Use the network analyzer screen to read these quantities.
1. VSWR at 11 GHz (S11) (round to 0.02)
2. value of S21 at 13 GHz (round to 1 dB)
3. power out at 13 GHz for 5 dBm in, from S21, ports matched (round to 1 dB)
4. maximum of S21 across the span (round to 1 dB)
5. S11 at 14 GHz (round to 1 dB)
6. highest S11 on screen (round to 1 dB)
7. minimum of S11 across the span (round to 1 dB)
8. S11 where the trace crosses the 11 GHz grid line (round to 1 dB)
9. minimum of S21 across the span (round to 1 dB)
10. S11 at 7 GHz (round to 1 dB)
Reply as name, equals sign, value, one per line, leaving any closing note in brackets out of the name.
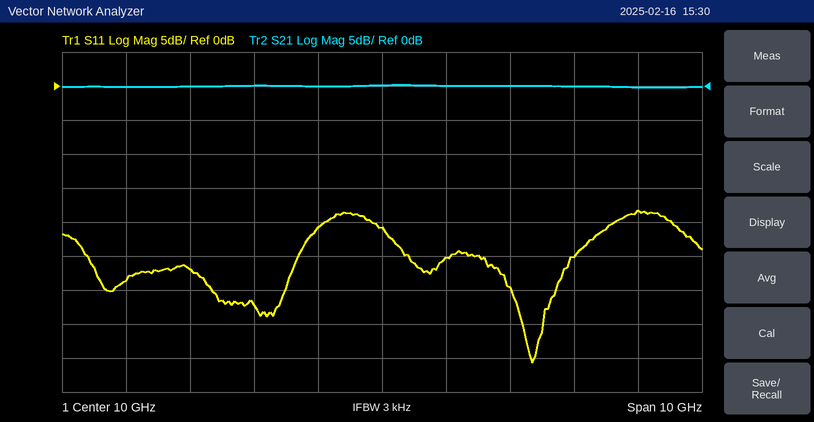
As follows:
VSWR at 11 GHz (S11) = 1.12
value of S21 at 13 GHz = 0 dB
power out at 13 GHz for 5 dBm in, from S21, ports matched = 5 dBm
maximum of S21 across the span = 0 dB
S11 at 14 GHz = -18 dB
highest S11 on screen = -18 dB
minimum of S11 across the span = -41 dB
S11 where the trace crosses the 11 GHz grid line = -25 dB
minimum of S21 across the span = 0 dB
S11 at 7 GHz = -27 dB
